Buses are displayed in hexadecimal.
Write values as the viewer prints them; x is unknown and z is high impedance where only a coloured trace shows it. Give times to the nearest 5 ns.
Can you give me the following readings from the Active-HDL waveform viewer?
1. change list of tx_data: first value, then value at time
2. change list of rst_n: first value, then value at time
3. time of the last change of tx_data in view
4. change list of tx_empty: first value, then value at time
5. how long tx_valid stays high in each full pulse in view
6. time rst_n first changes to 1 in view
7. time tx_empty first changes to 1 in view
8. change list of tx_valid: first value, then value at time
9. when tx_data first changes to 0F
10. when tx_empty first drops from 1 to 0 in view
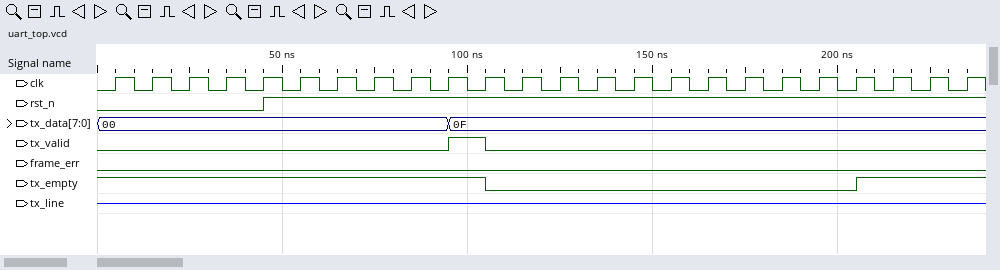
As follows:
00, 0F at 95 ns
0, 1 at 45 ns
95 ns
1, 0 at 105 ns, 1 at 205 ns
10 ns
45 ns
205 ns
0, 1 at 95 ns, 0 at 105 ns
95 ns
105 ns
